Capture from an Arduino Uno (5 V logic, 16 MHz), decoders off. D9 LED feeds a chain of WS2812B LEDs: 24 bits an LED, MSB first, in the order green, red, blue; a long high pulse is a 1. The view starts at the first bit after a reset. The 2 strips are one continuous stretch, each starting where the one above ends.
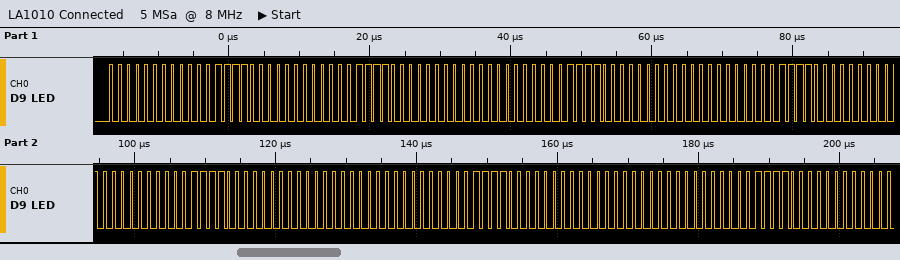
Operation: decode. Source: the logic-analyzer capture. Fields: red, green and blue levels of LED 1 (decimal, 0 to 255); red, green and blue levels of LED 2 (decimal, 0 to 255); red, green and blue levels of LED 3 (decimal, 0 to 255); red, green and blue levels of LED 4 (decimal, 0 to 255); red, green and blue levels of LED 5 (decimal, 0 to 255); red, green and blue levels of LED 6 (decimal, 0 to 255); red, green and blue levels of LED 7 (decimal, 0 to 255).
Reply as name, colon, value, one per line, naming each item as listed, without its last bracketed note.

red, green and blue levels of LED 1: 15, 0, 0
red, green and blue levels of LED 2: 0, 15, 0
red, green and blue levels of LED 3: 0, 15, 0
red, green and blue levels of LED 4: 0, 15, 0
red, green and blue levels of LED 5: 0, 15, 0
red, green and blue levels of LED 6: 15, 0, 0
red, green and blue levels of LED 7: 0, 0, 15
